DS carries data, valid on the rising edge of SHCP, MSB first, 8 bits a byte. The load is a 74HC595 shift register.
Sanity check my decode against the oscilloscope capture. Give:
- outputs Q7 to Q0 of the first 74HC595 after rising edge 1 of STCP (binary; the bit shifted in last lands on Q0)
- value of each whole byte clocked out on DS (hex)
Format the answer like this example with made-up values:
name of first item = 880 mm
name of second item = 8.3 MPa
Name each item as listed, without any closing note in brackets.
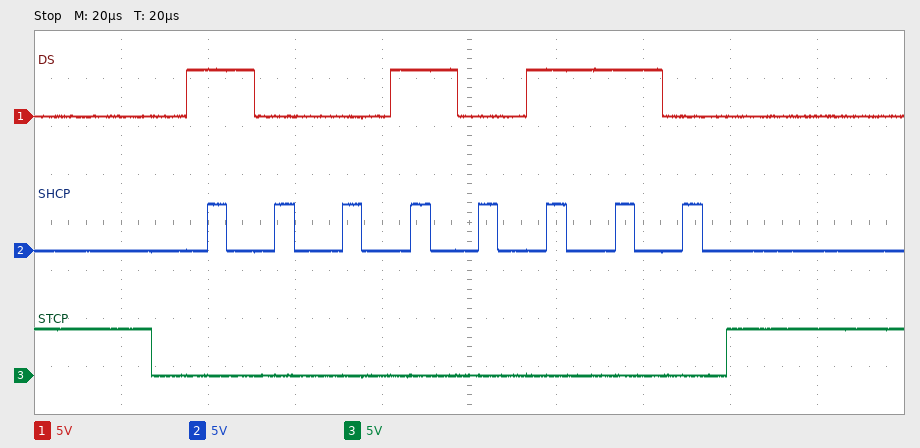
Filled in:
outputs Q7 to Q0 of the first 74HC595 after rising edge 1 of STCP = 10010110
value of each whole byte clocked out on DS = 0x96
